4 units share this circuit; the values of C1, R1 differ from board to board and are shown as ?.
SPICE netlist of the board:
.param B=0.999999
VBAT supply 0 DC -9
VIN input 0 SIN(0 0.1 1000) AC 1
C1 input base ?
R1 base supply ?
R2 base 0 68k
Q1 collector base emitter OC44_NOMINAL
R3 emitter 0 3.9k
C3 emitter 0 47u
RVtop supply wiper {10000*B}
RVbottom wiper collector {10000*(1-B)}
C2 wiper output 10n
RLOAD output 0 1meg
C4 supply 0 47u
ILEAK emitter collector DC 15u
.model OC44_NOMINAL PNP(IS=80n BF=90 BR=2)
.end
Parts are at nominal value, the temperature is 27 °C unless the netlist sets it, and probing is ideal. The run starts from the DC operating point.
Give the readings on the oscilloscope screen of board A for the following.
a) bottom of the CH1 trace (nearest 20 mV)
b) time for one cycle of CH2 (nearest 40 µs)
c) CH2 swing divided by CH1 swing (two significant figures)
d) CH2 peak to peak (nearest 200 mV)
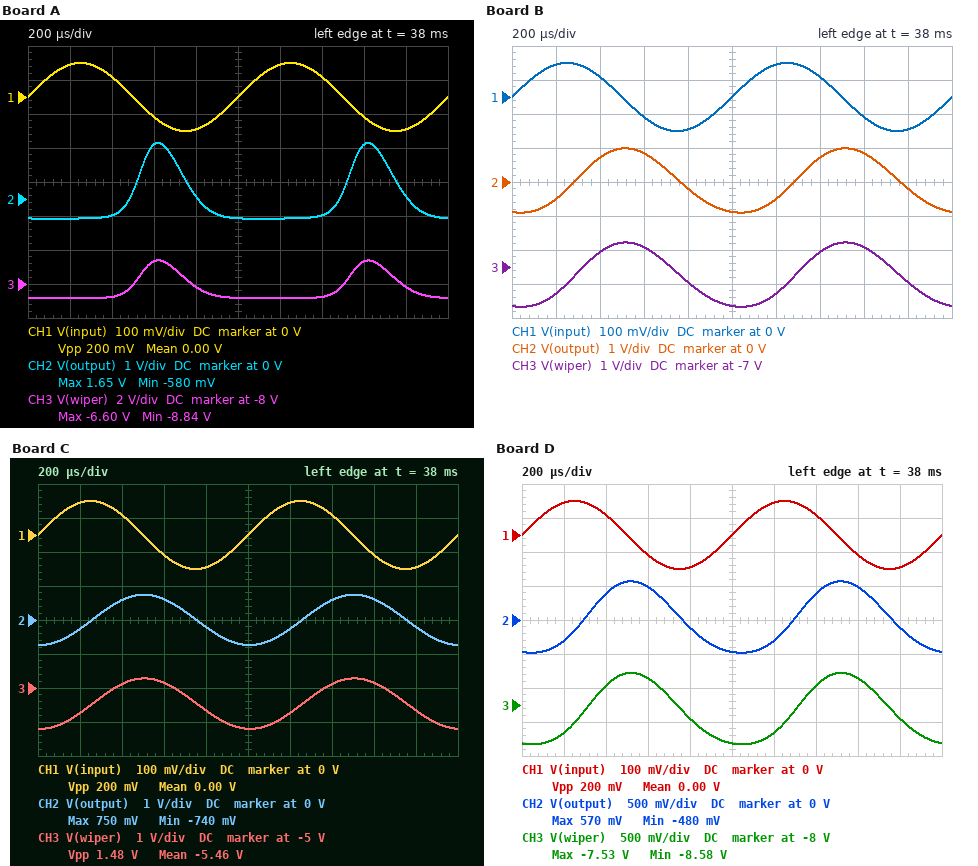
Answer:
-100 mV
1.00 ms
11
2.2 V
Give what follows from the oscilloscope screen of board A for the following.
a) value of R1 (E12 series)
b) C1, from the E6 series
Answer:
1.5 MΩ
6.8 nF
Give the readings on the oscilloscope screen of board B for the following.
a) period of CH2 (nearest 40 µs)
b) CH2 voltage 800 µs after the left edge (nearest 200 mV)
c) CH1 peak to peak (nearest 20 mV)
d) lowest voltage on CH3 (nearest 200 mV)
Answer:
1.00 ms
-200 mV
200 mV
-8.2 V
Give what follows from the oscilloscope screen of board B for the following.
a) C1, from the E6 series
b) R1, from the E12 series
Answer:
2.2 nF
560 kΩ
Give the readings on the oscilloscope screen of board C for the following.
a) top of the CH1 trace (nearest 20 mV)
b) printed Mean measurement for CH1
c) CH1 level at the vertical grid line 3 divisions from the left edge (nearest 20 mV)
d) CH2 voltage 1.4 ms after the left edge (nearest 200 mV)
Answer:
100 mV
0.00 V
-60 mV
600 mV
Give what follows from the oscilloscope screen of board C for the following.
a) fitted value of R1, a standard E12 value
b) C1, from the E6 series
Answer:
270 kΩ
1.5 nF
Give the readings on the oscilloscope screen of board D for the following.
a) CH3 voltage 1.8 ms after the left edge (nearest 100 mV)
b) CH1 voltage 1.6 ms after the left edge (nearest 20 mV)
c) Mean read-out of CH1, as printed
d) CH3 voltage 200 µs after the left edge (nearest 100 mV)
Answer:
-8.2 V
-60 mV
0.00 V
-8.4 V
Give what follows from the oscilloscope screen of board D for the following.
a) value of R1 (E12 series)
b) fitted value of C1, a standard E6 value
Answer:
1 MΩ
1.5 nF
